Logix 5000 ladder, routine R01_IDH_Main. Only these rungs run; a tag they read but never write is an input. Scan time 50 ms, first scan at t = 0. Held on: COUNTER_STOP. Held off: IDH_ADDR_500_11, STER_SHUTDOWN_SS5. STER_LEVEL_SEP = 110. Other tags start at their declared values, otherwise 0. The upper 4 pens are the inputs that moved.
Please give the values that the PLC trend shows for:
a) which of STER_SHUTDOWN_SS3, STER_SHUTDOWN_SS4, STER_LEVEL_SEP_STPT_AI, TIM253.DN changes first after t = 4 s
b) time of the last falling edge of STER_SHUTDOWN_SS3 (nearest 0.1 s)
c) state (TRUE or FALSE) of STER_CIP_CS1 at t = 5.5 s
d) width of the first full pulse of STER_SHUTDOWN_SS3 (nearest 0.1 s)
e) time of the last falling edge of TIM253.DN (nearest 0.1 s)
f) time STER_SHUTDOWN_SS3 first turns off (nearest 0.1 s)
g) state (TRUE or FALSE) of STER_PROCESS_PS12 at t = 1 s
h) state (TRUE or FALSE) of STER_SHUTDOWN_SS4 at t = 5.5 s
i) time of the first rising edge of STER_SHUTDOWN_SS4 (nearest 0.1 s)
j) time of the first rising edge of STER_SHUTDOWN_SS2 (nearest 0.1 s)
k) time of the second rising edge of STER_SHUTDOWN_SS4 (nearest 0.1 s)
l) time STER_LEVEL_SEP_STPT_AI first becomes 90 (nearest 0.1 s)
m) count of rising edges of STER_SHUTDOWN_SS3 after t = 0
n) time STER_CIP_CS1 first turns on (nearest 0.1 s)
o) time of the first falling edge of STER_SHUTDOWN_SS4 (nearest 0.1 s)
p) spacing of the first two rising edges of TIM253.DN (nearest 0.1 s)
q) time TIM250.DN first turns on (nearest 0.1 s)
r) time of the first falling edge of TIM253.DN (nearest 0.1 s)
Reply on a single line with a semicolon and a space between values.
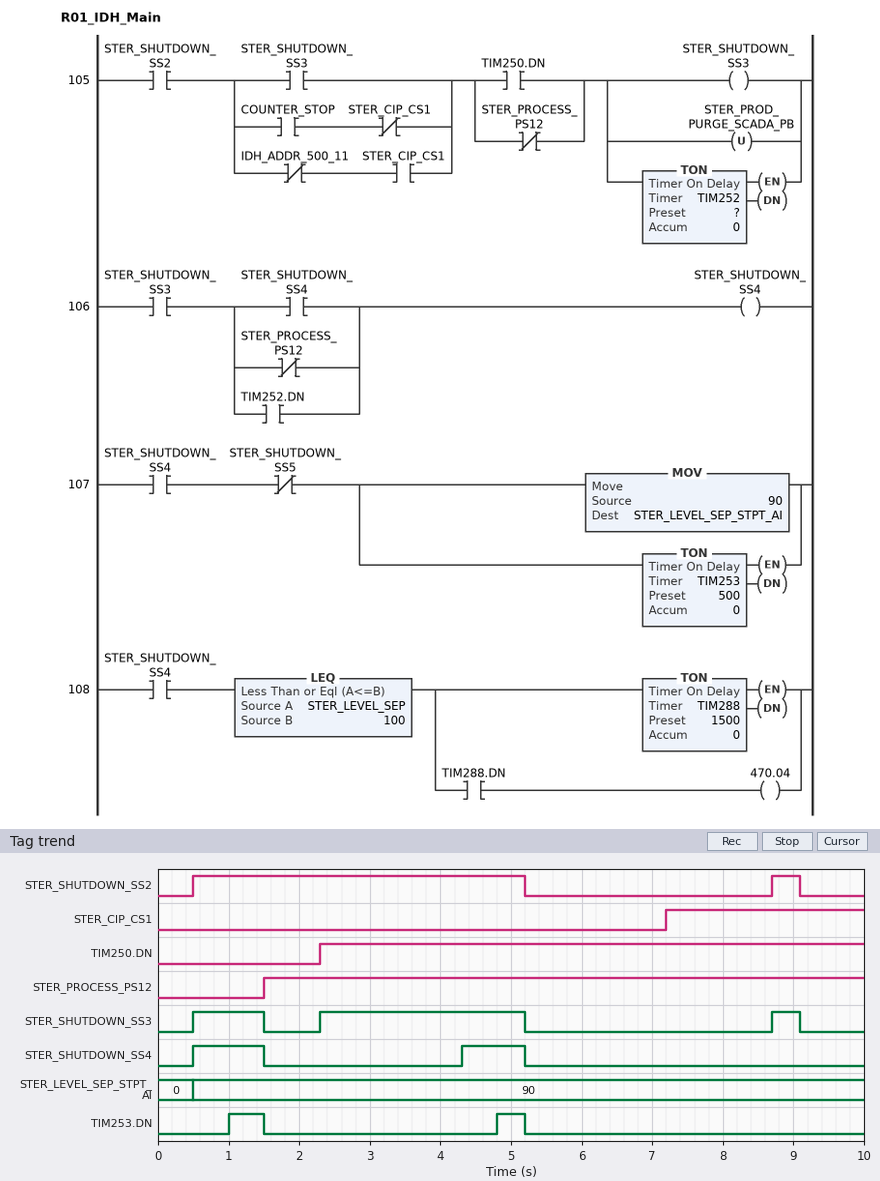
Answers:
STER_SHUTDOWN_SS4; 9.1 s; FALSE; 1.0 s; 5.2 s; 1.5 s; FALSE; FALSE; 0.5 s; 0.5 s; 4.3 s; 0.5 s; 3; 7.2 s; 1.5 s; 3.8 s; 2.3 s; 1.5 s
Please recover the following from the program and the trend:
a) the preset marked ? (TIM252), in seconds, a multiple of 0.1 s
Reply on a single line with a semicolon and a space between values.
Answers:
2.0 s
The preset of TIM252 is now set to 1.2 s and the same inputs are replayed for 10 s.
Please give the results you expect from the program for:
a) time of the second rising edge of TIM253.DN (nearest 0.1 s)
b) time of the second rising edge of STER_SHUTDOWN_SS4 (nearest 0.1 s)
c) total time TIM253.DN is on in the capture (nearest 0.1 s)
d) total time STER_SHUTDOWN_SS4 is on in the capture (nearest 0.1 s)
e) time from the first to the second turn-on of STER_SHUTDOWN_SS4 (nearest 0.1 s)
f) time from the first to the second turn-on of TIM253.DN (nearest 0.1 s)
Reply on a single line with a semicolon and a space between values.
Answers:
4.0 s; 3.5 s; 1.7 s; 2.7 s; 3.0 s; 3.0 s
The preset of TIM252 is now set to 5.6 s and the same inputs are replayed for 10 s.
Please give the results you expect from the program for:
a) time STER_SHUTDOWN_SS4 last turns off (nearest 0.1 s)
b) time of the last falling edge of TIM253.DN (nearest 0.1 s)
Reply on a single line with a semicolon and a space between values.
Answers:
1.5 s; 1.5 s
